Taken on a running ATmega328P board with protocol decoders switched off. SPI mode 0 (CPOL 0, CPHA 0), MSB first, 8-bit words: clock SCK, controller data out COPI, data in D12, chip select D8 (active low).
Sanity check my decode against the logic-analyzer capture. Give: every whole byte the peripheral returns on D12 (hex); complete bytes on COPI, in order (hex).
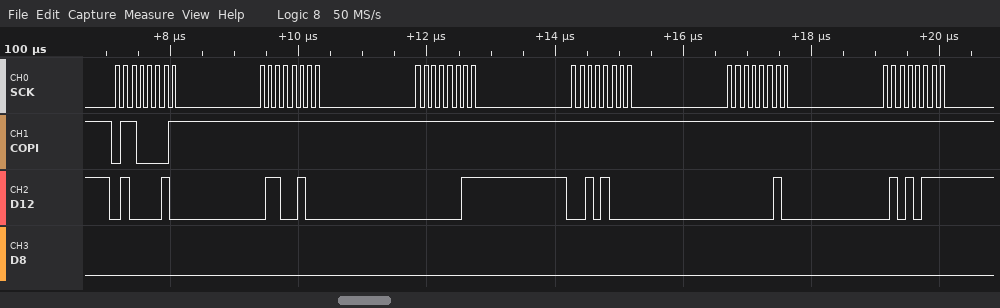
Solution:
42 64 03 28 02 57
61 FF FF FF FF FF
